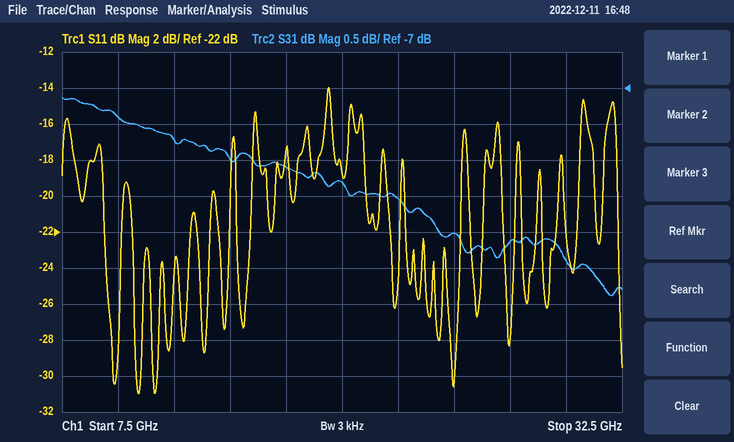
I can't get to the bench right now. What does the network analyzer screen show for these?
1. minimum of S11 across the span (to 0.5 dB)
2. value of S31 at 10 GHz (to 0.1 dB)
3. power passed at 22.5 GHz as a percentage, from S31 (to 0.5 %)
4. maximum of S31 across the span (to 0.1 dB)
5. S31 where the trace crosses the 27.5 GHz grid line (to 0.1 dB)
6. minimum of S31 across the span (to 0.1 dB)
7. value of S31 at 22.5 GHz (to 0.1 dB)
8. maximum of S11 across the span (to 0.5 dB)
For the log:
-31.0 dB
-7.4 dB
14.0 %
-7.1 dB
-9.1 dB
-9.9 dB
-8.5 dB
-14.0 dB
